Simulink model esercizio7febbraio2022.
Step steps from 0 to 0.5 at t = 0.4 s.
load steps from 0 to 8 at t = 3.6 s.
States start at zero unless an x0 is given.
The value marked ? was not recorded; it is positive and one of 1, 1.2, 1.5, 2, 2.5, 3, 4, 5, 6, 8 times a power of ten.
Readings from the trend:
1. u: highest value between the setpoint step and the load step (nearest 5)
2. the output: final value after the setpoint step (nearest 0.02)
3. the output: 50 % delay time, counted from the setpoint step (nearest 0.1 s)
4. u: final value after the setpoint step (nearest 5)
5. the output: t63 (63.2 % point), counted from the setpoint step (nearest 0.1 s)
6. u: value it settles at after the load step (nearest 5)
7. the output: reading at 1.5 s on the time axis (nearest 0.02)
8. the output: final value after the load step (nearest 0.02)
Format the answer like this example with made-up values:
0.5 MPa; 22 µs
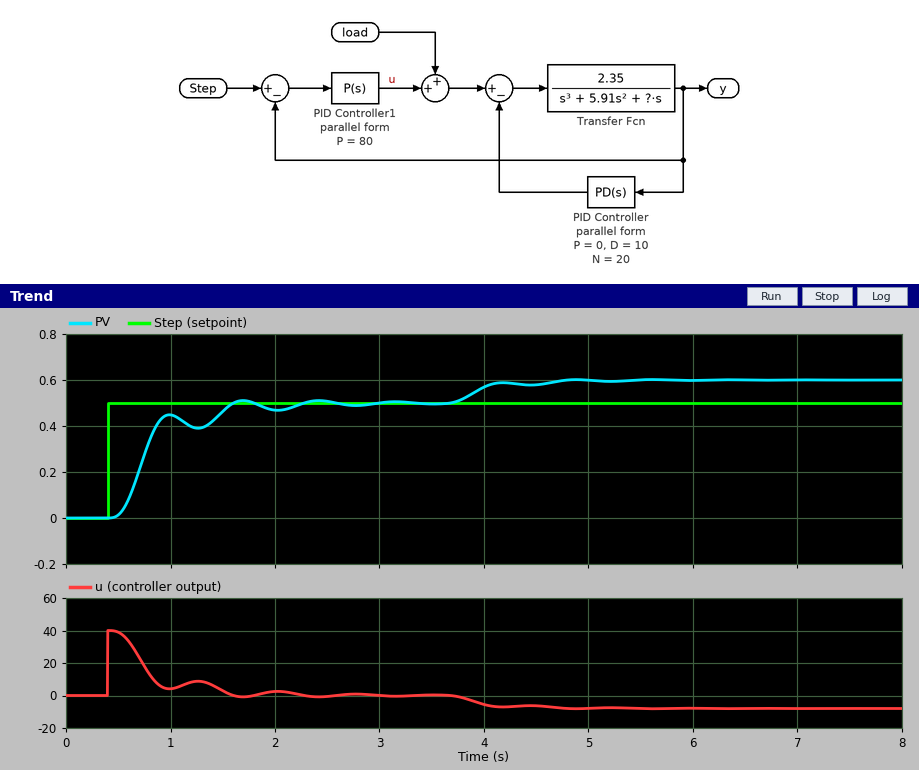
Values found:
40; 0.50; 0.3 s; 0; 0.4 s; -10; 0.46; 0.60
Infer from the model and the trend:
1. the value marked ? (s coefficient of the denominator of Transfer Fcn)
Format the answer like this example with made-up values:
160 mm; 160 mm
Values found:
60
